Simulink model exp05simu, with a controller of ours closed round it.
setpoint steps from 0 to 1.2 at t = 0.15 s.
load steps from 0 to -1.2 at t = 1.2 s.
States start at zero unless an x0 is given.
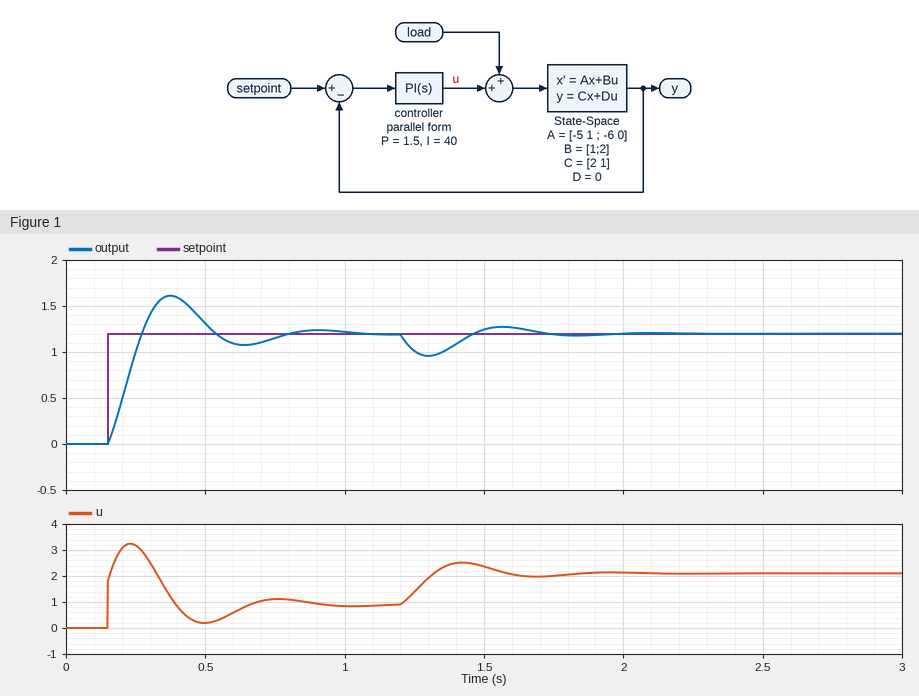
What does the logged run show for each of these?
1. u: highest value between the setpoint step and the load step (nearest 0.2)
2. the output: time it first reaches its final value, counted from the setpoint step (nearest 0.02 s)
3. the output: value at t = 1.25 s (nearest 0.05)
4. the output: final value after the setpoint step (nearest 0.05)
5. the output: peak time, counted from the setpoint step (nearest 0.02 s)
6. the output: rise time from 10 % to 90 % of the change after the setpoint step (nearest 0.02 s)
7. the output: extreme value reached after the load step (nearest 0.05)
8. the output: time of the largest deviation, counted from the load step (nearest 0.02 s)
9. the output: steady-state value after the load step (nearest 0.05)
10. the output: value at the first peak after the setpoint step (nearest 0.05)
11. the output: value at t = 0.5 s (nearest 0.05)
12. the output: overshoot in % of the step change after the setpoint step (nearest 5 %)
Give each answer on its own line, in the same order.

3.2
0.12 s
1.00
1.20
0.22 s
0.10 s
0.95
0.10 s
1.20
1.60
1.30
35 %
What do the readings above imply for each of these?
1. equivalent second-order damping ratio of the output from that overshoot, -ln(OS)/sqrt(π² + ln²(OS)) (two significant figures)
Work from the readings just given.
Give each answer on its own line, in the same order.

0.32
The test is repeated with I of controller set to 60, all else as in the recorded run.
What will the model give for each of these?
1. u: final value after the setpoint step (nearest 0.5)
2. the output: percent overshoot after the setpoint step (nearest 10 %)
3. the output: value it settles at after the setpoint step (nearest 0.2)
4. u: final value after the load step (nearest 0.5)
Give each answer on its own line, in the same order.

1.0
40 %
1.2
2.0
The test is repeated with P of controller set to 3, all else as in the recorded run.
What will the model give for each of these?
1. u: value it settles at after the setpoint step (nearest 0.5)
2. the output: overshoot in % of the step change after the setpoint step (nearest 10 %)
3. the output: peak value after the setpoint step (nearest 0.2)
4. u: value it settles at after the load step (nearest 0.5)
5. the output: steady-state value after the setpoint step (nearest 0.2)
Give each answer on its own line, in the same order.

1.0
20 %
1.4
2.0
1.2
